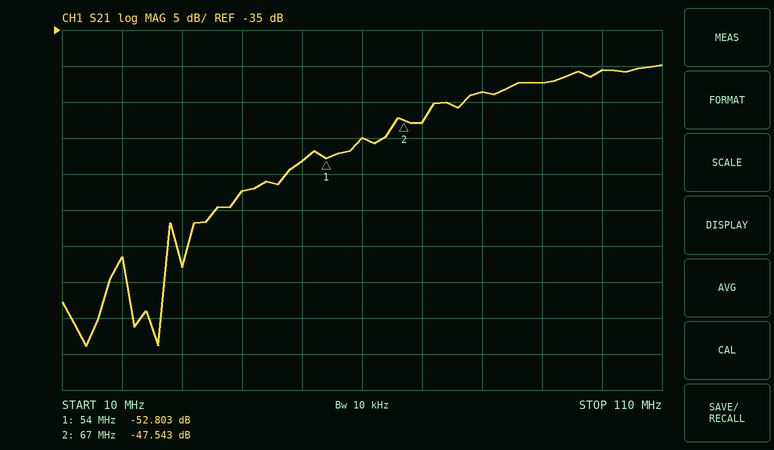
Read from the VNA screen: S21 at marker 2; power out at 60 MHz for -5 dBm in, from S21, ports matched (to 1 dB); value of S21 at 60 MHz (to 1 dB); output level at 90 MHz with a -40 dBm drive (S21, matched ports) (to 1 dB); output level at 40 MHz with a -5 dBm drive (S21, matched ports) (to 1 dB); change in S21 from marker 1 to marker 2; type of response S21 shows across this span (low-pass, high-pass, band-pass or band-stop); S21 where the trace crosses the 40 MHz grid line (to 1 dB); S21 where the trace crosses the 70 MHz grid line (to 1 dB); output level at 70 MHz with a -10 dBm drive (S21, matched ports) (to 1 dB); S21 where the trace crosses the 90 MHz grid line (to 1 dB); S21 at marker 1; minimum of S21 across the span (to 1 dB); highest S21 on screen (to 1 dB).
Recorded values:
-47.543 dB
-55 dBm
-50 dB
-82 dBm
-62 dBm
5.260 dB
high-pass
-57 dB
-48 dB
-58 dBm
-42 dB
-52.803 dB
-79 dB
-40 dB
